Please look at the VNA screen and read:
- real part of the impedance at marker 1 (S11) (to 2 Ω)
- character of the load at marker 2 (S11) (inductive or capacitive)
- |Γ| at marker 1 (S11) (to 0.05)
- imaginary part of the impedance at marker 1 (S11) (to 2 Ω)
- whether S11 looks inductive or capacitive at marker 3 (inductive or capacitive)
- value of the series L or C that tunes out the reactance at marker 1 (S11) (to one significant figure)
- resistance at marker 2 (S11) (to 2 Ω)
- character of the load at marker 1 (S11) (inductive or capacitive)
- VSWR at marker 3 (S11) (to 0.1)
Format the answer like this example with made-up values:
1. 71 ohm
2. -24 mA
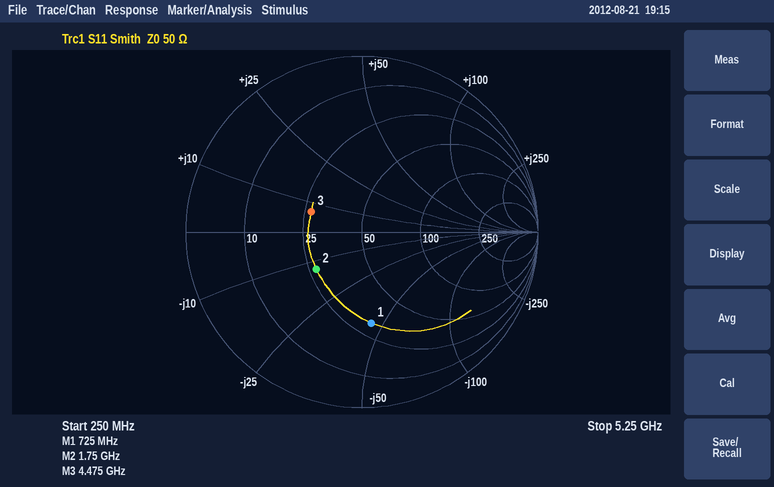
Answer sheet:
1. 32 Ω
2. capacitive
3. 0.50
4. -44 Ω
5. inductive
6. 10 nH
7. 28 Ω
8. capacitive
9. 1.9
